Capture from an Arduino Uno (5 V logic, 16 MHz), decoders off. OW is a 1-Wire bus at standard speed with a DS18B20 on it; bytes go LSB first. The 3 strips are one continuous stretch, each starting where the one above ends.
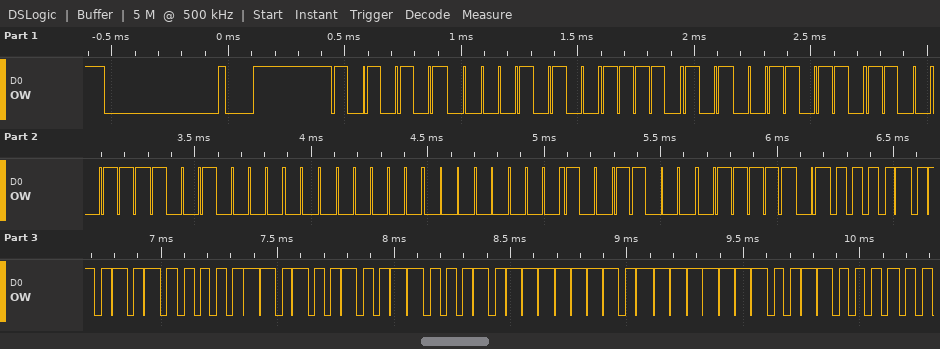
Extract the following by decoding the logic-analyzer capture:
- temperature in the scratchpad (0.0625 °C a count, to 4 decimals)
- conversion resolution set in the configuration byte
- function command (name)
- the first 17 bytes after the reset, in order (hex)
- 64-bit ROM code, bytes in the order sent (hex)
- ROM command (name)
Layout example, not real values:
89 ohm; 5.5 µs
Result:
85.0000 °C; 12 bits; Read Scratchpad; 55 28 AF 6C E3 09 00 00 19 BE 50 05 4B 46 7F FF 0C; 28 AF 6C E3 09 00 00 19; Match ROM
